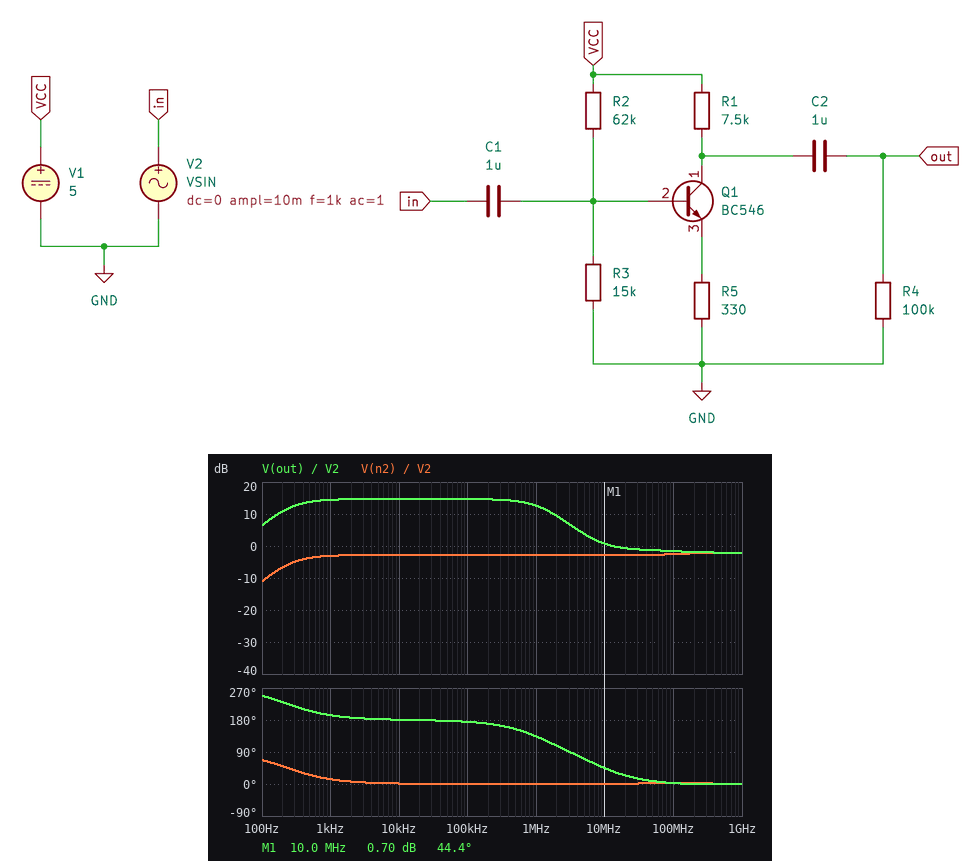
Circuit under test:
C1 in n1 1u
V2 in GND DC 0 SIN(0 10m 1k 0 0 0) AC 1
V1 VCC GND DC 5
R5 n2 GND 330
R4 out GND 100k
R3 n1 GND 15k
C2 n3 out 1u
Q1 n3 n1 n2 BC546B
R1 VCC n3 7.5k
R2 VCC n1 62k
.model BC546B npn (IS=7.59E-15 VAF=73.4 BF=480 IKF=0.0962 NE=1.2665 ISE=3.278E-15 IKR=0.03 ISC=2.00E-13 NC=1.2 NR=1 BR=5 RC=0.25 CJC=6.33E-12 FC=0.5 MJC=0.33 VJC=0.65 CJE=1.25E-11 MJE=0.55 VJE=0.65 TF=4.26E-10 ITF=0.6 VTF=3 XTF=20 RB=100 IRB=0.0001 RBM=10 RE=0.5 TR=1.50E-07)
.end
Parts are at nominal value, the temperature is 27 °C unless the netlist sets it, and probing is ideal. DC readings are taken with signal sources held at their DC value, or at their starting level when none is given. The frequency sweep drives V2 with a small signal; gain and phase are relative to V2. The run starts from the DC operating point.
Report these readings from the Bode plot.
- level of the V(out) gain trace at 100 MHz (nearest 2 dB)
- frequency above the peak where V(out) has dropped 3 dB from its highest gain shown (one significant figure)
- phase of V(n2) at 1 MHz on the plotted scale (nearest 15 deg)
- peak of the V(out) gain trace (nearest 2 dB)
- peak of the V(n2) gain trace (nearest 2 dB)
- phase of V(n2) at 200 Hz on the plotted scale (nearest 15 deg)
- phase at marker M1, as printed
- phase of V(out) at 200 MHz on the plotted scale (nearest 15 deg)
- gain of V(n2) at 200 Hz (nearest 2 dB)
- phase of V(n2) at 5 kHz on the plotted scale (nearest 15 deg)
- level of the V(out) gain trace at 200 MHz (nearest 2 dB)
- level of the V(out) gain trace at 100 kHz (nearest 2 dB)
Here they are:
-2 dB
1 MHz
0 deg
14 dB
-2 dB
45 deg
44.4 deg
0 deg
-6 dB
0 deg
-2 dB
14 dB
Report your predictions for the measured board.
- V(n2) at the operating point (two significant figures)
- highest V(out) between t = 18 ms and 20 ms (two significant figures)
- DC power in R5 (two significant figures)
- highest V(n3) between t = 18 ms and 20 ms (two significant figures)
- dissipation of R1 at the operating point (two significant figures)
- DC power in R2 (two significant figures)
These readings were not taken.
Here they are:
210 mV
160 mV
130 µW
490 mV
2.9 mW
280 µW
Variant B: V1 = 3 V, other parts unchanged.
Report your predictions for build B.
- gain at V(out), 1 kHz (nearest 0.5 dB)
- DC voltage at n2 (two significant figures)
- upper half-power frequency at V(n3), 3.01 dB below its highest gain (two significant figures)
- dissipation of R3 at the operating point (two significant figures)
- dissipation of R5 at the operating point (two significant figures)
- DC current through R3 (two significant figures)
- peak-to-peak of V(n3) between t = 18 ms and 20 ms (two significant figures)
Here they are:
15.5 dB
10 mV
5.3 MHz
23 µW
320 nW
39 µA
120 mV
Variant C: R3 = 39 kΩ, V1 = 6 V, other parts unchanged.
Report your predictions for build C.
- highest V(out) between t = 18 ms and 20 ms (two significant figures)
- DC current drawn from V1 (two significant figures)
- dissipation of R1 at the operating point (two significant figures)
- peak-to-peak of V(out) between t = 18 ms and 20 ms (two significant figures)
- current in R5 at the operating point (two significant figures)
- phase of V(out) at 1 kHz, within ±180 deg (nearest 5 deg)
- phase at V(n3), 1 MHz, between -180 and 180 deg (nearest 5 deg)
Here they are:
5.0 mV
840 µA
4.3 mW
6.3 mV
810 µA
-160 deg
55 deg
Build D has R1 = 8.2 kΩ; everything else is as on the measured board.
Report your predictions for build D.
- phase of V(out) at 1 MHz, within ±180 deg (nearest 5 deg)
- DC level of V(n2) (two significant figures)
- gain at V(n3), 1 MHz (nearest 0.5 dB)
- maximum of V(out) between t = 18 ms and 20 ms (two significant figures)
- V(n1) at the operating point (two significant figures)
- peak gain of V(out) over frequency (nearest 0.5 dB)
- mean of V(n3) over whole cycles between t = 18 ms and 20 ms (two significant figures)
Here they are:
130 deg
190 mV
11.0 dB
140 mV
840 mV
13.0 dB
340 mV
